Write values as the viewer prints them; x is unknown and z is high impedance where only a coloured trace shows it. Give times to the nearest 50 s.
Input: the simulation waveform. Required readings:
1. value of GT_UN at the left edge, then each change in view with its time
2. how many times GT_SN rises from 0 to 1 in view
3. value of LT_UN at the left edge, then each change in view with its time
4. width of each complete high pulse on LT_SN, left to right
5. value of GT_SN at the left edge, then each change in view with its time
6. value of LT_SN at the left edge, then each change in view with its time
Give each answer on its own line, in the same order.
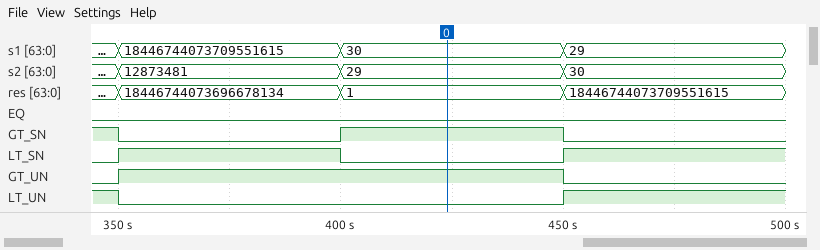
0, 1 at 350 s, 0 at 450 s
1
1, 0 at 350 s, 1 at 450 s
50 s
1, 0 at 350 s, 1 at 400 s, 0 at 450 s
0, 1 at 350 s, 0 at 400 s, 1 at 450 s
